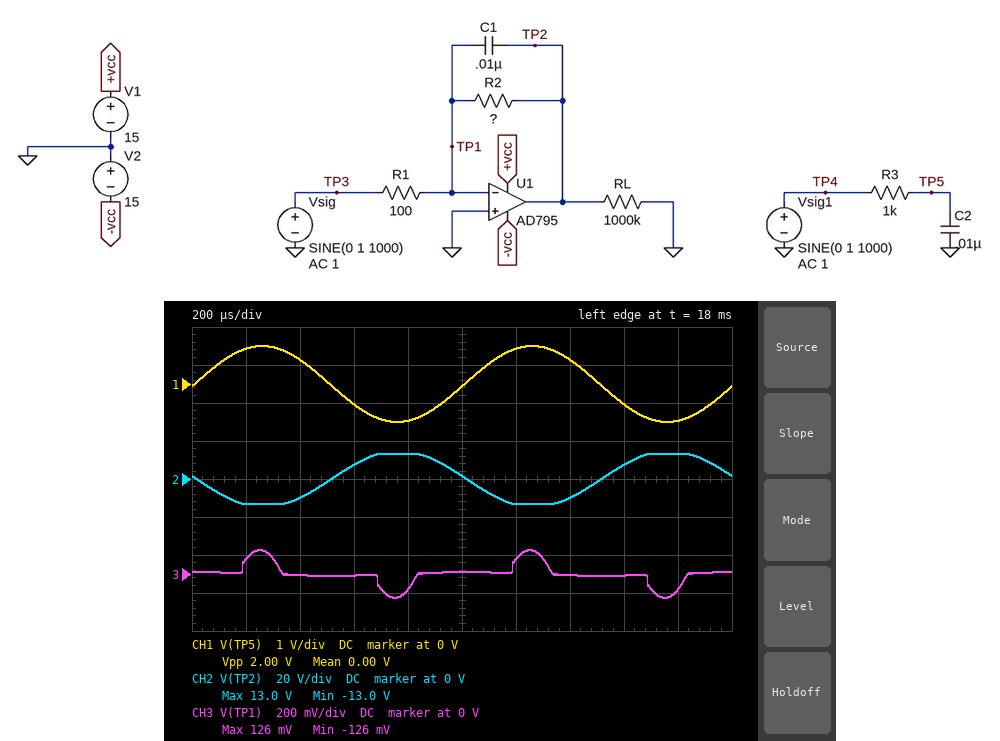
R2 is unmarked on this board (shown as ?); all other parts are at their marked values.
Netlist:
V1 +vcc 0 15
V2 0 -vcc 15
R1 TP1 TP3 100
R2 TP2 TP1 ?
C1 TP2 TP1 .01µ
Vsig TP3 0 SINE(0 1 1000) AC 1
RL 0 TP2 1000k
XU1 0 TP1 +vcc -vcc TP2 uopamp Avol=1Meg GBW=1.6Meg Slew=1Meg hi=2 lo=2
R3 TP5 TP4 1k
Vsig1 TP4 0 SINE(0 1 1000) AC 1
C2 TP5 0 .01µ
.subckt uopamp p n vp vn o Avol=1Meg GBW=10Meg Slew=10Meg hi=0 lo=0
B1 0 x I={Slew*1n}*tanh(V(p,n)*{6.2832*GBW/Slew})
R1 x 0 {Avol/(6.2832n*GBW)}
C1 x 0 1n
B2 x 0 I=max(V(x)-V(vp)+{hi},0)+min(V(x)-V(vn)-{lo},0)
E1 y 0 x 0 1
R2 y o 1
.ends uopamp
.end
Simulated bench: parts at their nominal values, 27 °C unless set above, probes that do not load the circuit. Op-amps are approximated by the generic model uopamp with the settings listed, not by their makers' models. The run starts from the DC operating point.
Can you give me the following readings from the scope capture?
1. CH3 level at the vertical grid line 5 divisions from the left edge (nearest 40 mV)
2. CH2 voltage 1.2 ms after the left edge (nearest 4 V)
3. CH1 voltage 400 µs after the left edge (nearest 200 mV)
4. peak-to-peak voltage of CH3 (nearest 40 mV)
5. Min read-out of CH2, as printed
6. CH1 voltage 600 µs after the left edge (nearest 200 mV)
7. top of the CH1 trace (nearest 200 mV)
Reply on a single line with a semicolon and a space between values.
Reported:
0 V; -12 V; 600 mV; 240 mV; -13.0 V; -600 mV; 1.0 V
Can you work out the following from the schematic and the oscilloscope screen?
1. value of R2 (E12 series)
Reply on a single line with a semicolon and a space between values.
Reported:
1.5 kΩ
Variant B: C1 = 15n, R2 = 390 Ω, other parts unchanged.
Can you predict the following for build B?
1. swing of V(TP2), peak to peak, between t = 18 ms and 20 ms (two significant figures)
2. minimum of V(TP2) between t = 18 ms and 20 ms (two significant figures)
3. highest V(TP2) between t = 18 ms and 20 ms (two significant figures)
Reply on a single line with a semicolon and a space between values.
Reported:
7.8 V; -3.9 V; 3.9 V
